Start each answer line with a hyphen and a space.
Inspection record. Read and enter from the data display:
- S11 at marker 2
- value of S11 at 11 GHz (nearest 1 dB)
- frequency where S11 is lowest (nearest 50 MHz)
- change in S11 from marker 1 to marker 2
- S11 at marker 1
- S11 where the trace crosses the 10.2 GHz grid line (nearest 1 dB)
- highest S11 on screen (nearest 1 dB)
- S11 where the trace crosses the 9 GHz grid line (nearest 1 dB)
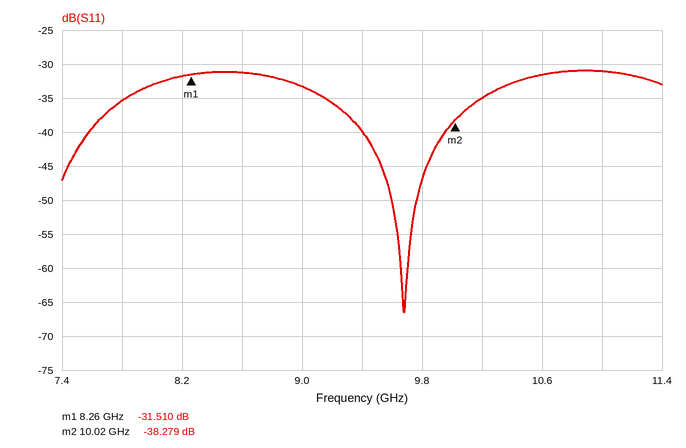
- -38.279 dB
- -31 dB
- 9.70 GHz
- -6.769 dB
- -31.510 dB
- -35 dB
- -31 dB
- -33 dB
